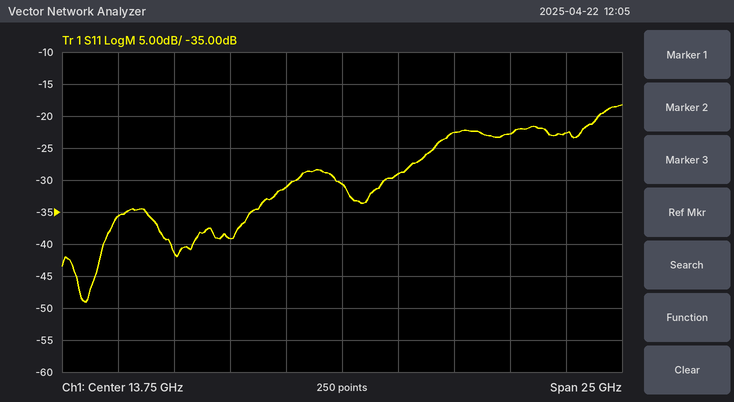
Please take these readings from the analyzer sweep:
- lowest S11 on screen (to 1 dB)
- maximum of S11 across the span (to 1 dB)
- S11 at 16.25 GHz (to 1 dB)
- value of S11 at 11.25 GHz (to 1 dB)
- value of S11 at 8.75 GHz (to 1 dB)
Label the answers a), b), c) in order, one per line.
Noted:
a) -49 dB
b) -18 dB
c) -29 dB
d) -31 dB
e) -39 dB
